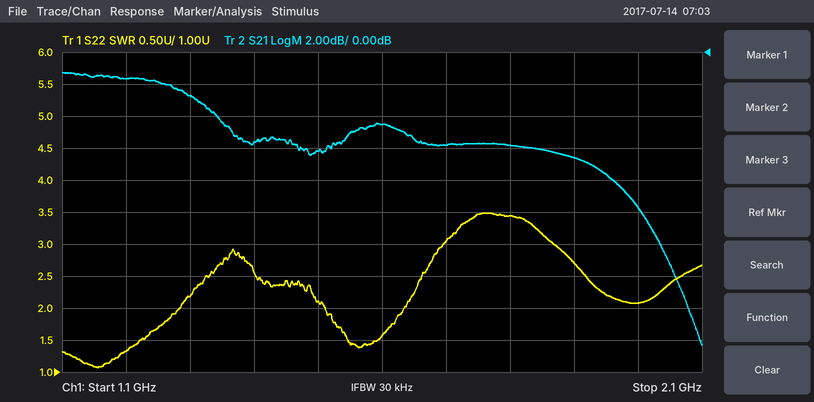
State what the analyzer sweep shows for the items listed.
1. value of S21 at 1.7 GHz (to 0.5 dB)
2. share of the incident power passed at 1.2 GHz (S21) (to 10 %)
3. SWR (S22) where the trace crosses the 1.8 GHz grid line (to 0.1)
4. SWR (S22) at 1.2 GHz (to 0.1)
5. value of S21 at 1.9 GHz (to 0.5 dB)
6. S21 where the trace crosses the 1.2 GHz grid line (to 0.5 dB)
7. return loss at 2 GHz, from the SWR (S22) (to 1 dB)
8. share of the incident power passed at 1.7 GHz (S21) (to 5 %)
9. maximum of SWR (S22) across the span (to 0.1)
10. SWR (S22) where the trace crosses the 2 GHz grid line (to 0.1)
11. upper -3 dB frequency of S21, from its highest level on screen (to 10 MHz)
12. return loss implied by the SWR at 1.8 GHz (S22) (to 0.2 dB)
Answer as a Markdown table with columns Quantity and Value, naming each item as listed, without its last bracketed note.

| Quantity | Value |
|---|---|
| value of S21 at 1.7 GHz | -6.0 dB |
| share of the incident power passed at 1.2 GHz (S21) | 70 % |
| SWR (S22) where the trace crosses the 1.8 GHz grid line | 3.4 |
| SWR (S22) at 1.2 GHz | 1.3 |
| value of S21 at 1.9 GHz | -6.5 dB |
| S21 where the trace crosses the 1.2 GHz grid line | -1.5 dB |
| return loss at 2 GHz, from the SWR (S22) | 9 dB |
| share of the incident power passed at 1.7 GHz (S21) | 25 % |
| maximum of SWR (S22) across the span | 3.5 |
| SWR (S22) where the trace crosses the 2 GHz grid line | 2.1 |
| upper -3 dB frequency of S21, from its highest level on screen | 1.35 GHz |
| return loss implied by the SWR at 1.8 GHz (S22) | 5.2 dB |
